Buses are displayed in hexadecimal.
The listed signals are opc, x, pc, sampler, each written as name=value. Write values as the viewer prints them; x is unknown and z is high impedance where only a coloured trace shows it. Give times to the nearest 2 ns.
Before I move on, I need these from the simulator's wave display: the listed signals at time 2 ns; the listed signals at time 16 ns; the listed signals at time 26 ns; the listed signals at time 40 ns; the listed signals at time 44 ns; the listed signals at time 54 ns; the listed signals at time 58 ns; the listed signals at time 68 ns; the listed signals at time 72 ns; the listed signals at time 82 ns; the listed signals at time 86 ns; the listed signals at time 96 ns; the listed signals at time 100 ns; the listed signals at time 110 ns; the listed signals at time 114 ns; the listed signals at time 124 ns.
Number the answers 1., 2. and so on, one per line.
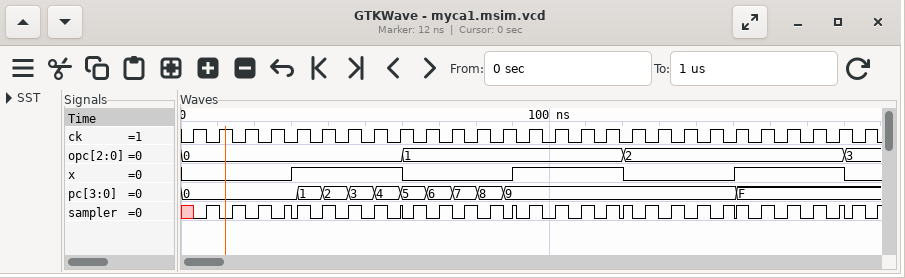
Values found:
1. opc=0, x=0, pc=0, sampler=x
2. opc=0, x=0, pc=0, sampler=1
3. opc=0, x=0, pc=0, sampler=0
4. opc=0, x=1, pc=2, sampler=1
5. opc=0, x=1, pc=2, sampler=0
6. opc=0, x=1, pc=4, sampler=1
7. opc=0, x=1, pc=4, sampler=0
8. opc=1, x=0, pc=6, sampler=0
9. opc=1, x=0, pc=6, sampler=1
10. opc=1, x=0, pc=8, sampler=0
11. opc=1, x=0, pc=8, sampler=1
12. opc=1, x=1, pc=9, sampler=1
13. opc=1, x=1, pc=9, sampler=0
14. opc=1, x=1, pc=9, sampler=1
15. opc=1, x=1, pc=9, sampler=0
16. opc=2, x=0, pc=9, sampler=0
